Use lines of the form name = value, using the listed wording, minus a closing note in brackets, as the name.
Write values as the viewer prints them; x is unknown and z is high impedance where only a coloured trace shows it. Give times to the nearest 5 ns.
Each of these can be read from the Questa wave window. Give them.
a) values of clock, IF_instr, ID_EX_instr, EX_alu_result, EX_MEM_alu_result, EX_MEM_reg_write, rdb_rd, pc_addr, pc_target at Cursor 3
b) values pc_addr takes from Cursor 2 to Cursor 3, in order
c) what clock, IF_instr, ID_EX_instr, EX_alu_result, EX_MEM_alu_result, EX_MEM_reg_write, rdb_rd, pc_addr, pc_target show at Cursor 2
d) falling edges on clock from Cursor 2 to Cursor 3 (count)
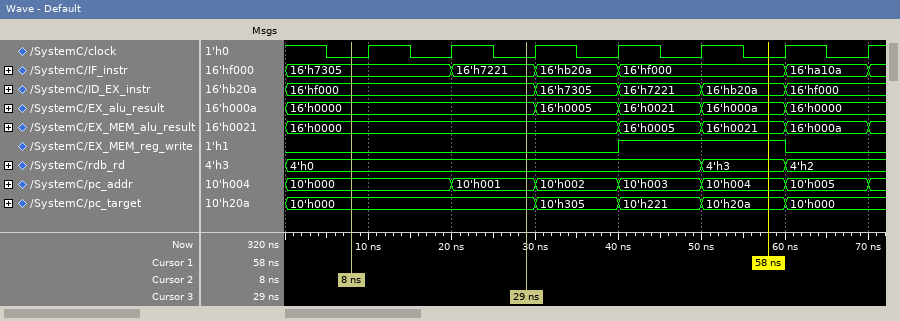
values of clock, IF_instr, ID_EX_instr, EX_alu_result, EX_MEM_alu_result, EX_MEM_reg_write, rdb_rd, pc_addr, pc_target at Cursor 3 = clock=0, IF_instr=16'h7221, ID_EX_instr=16'hf000, EX_alu_result=16'h0000, EX_MEM_alu_result=16'h0000, EX_MEM_reg_write=0, rdb_rd=4'h0, pc_addr=10'h001, pc_target=10'h000
values pc_addr takes from Cursor 2 to Cursor 3, in order = 10'h000, 10'h001
what clock, IF_instr, ID_EX_instr, EX_alu_result, EX_MEM_alu_result, EX_MEM_reg_write, rdb_rd, pc_addr, pc_target show at Cursor 2 = clock=0, IF_instr=16'h7305, ID_EX_instr=16'hf000, EX_alu_result=16'h0000, EX_MEM_alu_result=16'h0000, EX_MEM_reg_write=0, rdb_rd=4'h0, pc_addr=10'h000, pc_target=10'h000
falling edges on clock from Cursor 2 to Cursor 3 = 2
